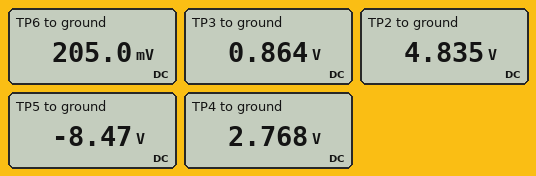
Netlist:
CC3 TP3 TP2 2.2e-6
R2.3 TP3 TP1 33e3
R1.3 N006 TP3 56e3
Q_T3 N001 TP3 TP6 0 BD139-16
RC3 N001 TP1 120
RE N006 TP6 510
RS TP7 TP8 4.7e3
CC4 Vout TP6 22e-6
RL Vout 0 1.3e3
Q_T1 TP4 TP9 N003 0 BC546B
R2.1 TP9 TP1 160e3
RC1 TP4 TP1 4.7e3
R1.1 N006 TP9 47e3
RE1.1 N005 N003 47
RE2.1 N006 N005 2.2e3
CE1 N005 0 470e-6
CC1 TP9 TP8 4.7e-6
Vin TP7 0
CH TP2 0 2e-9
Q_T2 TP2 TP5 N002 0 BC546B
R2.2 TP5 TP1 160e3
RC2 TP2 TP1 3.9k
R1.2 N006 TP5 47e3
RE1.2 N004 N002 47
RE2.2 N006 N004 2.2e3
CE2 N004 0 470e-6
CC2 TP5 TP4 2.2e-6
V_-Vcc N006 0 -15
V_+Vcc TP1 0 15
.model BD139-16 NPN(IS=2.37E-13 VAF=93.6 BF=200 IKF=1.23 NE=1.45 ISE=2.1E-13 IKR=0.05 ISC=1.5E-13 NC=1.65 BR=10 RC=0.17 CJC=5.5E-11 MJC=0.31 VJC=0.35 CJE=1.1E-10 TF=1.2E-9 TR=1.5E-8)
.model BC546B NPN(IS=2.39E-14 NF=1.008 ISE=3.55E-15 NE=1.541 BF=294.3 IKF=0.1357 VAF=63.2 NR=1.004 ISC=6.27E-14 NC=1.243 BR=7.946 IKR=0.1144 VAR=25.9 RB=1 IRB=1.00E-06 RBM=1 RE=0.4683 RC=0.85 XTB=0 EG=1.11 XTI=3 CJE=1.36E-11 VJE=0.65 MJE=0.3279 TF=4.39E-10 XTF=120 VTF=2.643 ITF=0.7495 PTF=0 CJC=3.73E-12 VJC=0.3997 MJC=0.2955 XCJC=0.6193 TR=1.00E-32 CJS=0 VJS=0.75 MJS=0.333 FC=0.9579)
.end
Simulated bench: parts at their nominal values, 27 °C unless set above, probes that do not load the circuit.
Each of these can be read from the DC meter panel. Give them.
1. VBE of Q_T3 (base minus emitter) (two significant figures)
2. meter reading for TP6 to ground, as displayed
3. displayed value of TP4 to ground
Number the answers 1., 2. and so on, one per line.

1. 660 mV
2. 205.0 mV
3. 2.768 V
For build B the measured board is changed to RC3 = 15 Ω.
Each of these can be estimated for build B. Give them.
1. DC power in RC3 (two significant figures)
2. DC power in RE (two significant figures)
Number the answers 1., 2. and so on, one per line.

1. 13 mW
2. 460 mW
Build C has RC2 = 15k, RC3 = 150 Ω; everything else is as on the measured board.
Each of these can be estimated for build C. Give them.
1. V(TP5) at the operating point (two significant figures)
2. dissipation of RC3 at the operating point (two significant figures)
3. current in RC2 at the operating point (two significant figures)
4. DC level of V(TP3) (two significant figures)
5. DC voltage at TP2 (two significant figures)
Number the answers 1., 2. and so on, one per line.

1. -10 V
2. 130 mW
3. 1.7 mA
4. 840 mV
5. -11 V
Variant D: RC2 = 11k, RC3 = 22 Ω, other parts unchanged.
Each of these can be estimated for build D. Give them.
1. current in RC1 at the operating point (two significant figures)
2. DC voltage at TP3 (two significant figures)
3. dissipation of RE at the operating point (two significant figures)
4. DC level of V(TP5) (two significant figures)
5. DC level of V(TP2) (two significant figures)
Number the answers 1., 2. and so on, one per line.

1. 2.6 mA
2. 930 mV
3. 460 mW
4. -9.2 V
5. -9.8 V
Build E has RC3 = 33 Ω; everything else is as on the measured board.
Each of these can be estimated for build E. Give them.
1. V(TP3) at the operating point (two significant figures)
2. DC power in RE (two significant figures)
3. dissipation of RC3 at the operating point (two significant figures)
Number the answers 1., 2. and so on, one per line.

1. 920 mV
2. 460 mW
3. 29 mW
